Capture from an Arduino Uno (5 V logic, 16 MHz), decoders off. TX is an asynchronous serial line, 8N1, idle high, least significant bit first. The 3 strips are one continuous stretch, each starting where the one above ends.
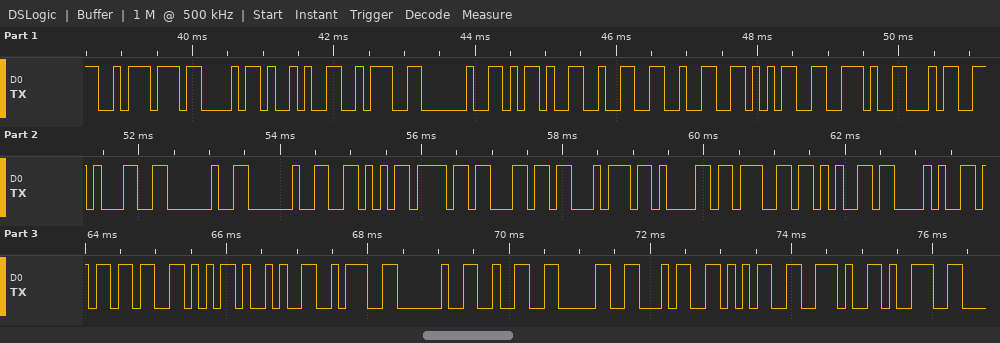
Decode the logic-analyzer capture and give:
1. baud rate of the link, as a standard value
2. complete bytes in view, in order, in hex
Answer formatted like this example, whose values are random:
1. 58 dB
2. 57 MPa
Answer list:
1. 9600 baud
2. BA 43 29 3A 20 2D 32 32 35 2E 34 31 20 20 56 6F 6C 74 61 67 65 28 6D 56 29 3A 20 32 30 34 35 2E 39
